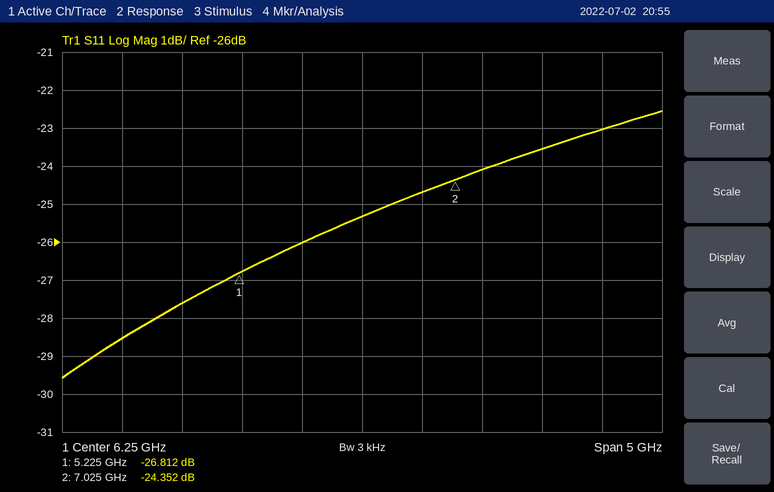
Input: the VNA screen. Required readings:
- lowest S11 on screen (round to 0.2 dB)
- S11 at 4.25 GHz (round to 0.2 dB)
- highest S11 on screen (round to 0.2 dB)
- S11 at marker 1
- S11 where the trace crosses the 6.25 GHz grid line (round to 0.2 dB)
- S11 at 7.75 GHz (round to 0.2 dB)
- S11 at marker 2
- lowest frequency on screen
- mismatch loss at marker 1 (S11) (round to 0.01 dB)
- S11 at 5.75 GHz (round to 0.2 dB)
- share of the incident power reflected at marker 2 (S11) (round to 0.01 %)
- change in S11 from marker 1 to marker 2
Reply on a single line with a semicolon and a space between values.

-29.6 dB; -28.6 dB; -22.6 dB; -26.812 dB; -25.4 dB; -23.6 dB; -24.352 dB; 3.75 GHz; 0.01 dB; -26.0 dB; 0.37 %; 2.460 dB
